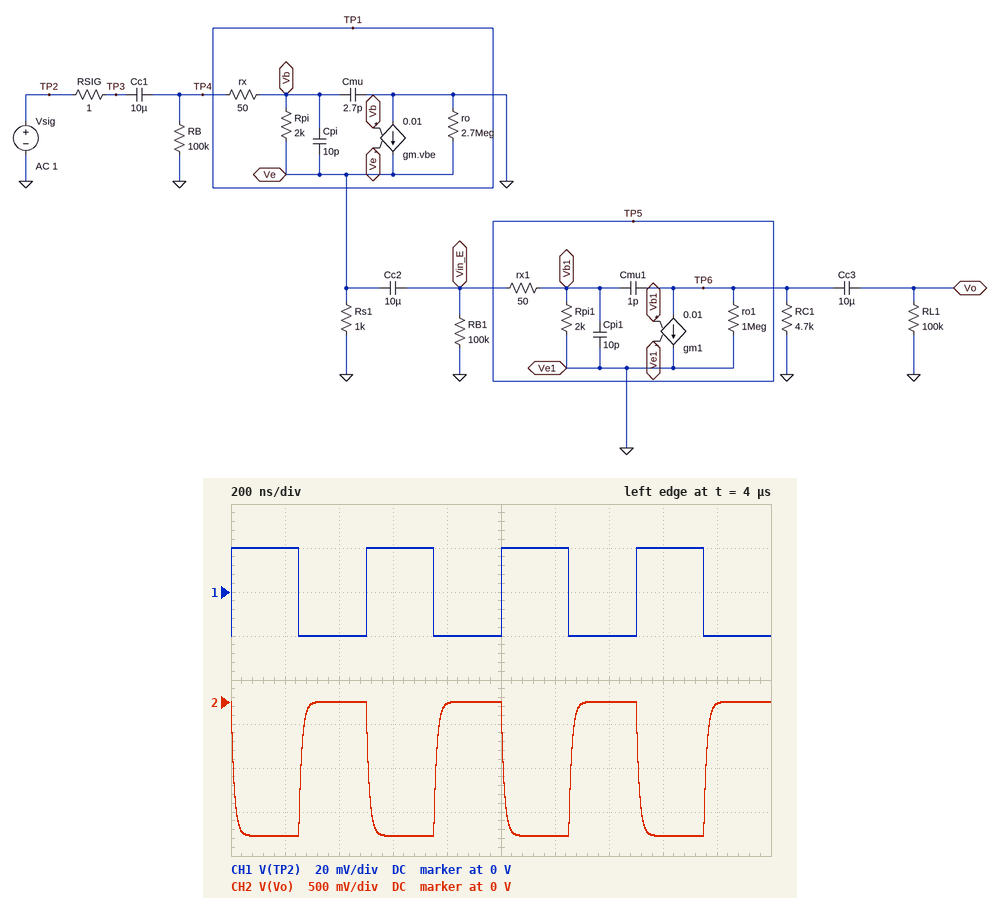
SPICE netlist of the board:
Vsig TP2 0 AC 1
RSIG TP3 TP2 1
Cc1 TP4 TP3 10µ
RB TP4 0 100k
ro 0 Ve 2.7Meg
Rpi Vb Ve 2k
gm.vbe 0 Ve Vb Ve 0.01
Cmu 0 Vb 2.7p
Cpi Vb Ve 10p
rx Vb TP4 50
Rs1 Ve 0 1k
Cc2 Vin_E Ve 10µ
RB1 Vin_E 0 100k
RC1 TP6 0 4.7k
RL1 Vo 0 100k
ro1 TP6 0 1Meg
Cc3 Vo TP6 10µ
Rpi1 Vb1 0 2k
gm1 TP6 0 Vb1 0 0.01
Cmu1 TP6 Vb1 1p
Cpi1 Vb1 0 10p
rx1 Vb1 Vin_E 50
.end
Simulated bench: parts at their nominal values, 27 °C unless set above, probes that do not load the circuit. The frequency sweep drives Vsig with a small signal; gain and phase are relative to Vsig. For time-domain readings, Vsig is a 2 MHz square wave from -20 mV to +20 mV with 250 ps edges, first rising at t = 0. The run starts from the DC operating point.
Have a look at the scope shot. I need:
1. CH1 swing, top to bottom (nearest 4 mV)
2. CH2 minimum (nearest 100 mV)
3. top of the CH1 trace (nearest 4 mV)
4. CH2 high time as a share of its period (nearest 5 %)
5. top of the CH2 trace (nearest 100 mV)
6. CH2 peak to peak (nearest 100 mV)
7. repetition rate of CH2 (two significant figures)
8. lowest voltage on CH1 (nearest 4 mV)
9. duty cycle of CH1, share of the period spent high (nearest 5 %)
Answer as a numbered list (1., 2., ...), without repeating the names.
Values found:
1. 40 mV
2. -1.5 V
3. 20 mV
4. 50 %
5. 0 V
6. 1.5 V
7. 2.0 MHz
8. -20 mV
9. 50 %
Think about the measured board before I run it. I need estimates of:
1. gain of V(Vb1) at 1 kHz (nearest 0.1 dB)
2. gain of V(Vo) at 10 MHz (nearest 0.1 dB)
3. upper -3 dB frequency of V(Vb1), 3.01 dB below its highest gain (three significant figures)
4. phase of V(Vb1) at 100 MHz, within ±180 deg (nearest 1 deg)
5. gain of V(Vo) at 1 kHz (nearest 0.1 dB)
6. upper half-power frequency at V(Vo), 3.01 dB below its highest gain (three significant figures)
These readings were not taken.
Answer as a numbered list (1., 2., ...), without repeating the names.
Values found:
1. -1.4 dB
2. 29.8 dB
3. 16.9 MHz
4. -27 deg
5. 31.6 dB
6. 14.0 MHz
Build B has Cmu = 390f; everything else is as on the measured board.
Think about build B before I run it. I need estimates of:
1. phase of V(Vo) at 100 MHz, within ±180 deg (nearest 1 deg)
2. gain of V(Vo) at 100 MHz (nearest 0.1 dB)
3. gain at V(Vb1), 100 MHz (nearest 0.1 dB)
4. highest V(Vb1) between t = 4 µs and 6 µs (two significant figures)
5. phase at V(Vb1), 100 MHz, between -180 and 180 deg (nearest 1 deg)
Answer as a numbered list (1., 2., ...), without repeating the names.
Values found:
1. 83 deg
2. 14.4 dB
3. -9.1 dB
4. 34 mV
5. -23 deg
